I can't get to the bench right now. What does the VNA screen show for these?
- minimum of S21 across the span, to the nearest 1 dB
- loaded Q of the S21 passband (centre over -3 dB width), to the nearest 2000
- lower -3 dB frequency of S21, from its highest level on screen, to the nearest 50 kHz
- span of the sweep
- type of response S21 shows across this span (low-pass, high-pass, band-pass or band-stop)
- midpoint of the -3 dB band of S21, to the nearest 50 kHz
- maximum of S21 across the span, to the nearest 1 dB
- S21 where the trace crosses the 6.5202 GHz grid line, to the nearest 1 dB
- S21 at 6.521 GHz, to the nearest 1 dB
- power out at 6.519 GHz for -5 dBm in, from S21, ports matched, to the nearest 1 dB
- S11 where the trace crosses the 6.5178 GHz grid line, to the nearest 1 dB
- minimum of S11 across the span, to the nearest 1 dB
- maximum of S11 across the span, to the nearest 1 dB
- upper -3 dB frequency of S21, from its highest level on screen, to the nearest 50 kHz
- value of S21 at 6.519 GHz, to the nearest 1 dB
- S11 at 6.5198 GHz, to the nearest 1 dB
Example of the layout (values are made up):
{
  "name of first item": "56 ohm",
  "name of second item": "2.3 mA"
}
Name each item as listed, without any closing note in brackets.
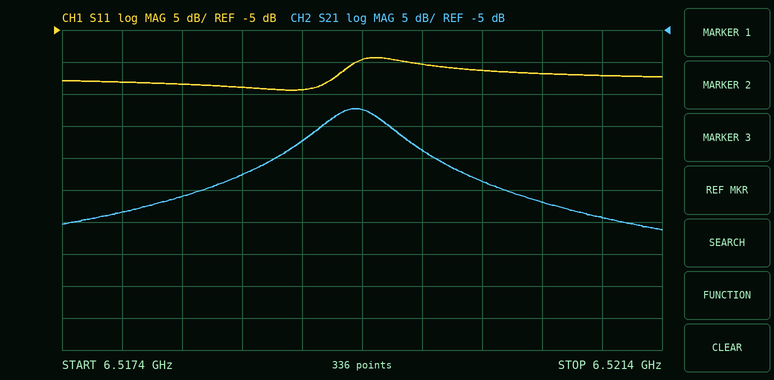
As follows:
{
  "minimum of S21 across the span, to the nearest 1 dB": "-36 dB",
  "loaded Q of the S21 passband (centre over -3 dB width), to the nearest 2000": "14000",
  "lower -3 dB frequency of S21, from its highest level on screen, to the nearest 50 kHz": "6.51910 GHz",
  "span of the sweep": "4 MHz",
  "type of response S21 shows across this span": "band-pass",
  "midpoint of the -3 dB band of S21, to the nearest 50 kHz": "6.51935 GHz",
  "maximum of S21 across the span, to the nearest 1 dB": "-17 dB",
  "S21 where the trace crosses the 6.5202 GHz grid line, to the nearest 1 dB": "-29 dB",
  "S21 at 6.521 GHz, to the nearest 1 dB": "-34 dB",
  "power out at 6.519 GHz for -5 dBm in, from S21, ports matched, to the nearest 1 dB": "-27 dBm",
  "S11 where the trace crosses the 6.5178 GHz grid line, to the nearest 1 dB": "-13 dB",
  "minimum of S11 across the span, to the nearest 1 dB": "-14 dB",
  "maximum of S11 across the span, to the nearest 1 dB": "-9 dB",
  "upper -3 dB frequency of S21, from its highest level on screen, to the nearest 50 kHz": "6.51960 GHz",
  "value of S21 at 6.519 GHz, to the nearest 1 dB": "-22 dB",
  "S11 at 6.5198 GHz, to the nearest 1 dB": "-10 dB"
}
